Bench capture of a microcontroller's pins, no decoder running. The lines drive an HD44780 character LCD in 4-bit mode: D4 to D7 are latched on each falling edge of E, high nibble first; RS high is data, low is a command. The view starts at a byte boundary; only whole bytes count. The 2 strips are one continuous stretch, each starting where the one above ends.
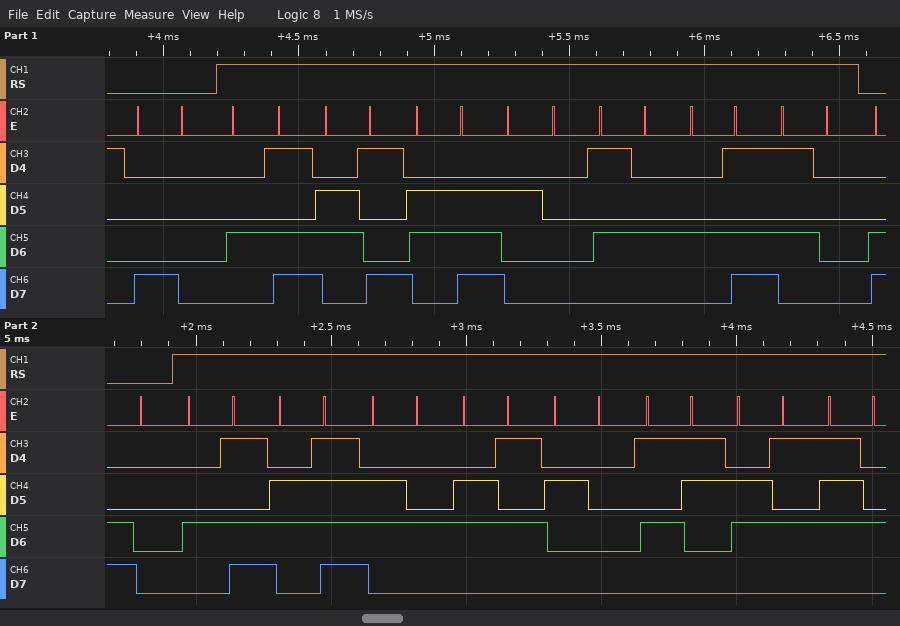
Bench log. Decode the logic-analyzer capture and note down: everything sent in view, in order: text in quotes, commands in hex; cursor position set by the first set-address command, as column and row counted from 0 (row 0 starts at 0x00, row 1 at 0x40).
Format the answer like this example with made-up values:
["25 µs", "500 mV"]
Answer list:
["0x80 \"Min TMP\" 0xC0 \"Mode Set\"", "column 0, row 0"]
